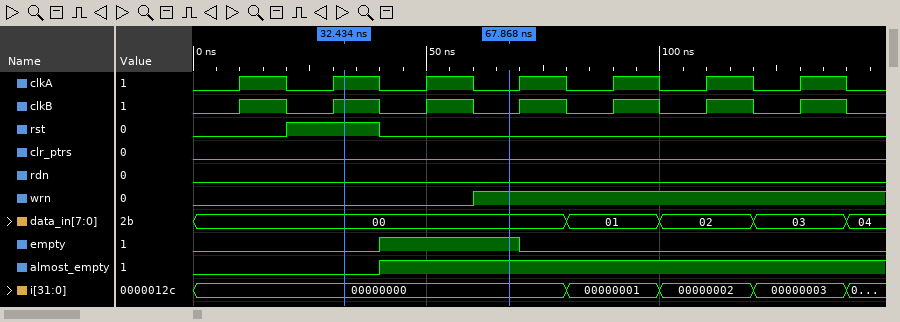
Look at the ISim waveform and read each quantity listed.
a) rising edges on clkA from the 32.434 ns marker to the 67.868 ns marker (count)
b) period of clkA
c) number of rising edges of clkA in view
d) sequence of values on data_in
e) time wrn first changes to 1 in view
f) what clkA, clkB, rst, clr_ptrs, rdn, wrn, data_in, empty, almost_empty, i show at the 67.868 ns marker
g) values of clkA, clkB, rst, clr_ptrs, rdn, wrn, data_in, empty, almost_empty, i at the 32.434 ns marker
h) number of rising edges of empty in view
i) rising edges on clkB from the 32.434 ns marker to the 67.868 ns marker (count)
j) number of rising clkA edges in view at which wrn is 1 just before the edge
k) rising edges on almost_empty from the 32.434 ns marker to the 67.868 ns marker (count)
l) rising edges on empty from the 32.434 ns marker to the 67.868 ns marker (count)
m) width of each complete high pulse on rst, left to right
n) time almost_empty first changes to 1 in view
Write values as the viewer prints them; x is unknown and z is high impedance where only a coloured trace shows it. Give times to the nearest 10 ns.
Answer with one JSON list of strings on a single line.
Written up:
["1", "20 ns", "7", "00, 01, 02, 03, 04", "60 ns", "clkA=0, clkB=0, rst=0, clr_ptrs=0, rdn=0, wrn=1, data_in=00, empty=1, almost_empty=1, i=00000000", "clkA=1, clkB=1, rst=1, clr_ptrs=0, rdn=0, wrn=0, data_in=00, empty=0, almost_empty=0, i=00000000", "1", "1", "4", "1", "1", "20 ns", "40 ns"]
